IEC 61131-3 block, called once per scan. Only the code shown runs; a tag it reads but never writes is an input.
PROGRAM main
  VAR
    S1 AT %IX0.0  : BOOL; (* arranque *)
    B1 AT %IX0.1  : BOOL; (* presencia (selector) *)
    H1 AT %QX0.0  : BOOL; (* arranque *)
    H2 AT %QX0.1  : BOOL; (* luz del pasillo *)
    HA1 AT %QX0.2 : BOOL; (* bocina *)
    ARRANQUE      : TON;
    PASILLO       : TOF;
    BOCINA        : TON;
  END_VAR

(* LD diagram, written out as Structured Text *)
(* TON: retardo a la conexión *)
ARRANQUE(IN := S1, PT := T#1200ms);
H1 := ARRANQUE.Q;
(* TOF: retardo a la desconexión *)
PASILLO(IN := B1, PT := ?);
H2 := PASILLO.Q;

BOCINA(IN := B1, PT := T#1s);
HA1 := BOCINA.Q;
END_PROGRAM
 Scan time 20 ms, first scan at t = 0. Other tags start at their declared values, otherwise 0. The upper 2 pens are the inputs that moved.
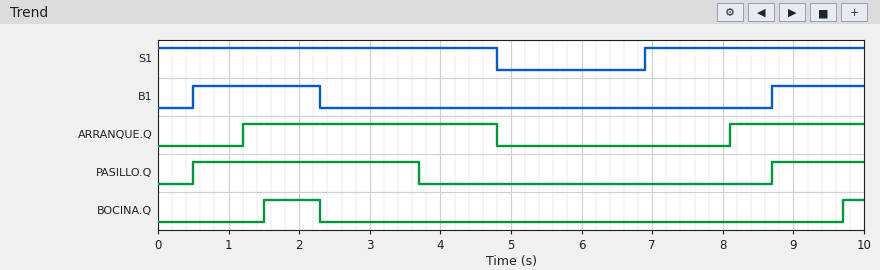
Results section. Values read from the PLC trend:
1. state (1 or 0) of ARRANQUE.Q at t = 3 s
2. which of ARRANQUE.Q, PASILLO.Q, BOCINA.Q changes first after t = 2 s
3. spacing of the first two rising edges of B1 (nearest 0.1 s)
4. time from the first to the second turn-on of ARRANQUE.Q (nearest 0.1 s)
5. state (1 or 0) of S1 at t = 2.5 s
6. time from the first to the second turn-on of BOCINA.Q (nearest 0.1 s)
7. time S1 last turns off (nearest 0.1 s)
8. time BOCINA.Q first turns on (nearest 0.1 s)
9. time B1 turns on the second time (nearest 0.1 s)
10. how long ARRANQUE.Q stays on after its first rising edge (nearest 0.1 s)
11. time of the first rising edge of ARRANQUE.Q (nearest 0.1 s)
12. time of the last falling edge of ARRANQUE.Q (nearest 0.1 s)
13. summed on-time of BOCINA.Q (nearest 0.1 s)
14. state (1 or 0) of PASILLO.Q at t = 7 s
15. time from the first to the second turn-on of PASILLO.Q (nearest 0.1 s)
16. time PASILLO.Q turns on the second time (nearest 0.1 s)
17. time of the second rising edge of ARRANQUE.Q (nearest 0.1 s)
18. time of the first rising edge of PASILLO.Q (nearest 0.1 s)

1
BOCINA.Q
8.2 s
6.9 s
1
8.2 s
4.8 s
1.5 s
8.7 s
3.6 s
1.2 s
4.8 s
1.1 s
0
8.2 s
8.7 s
8.1 s
0.5 s
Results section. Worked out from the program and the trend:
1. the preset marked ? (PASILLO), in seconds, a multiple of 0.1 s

1.4 s
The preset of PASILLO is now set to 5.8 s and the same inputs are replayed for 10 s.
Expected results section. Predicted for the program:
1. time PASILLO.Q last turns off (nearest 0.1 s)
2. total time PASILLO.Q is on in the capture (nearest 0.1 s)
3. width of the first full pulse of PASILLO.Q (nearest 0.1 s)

8.1 s
8.9 s
7.6 s
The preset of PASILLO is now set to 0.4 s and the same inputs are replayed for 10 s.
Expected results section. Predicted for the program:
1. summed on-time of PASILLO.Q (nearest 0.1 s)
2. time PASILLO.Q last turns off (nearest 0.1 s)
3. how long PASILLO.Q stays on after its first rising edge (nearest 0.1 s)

3.5 s
2.7 s
2.2 s
